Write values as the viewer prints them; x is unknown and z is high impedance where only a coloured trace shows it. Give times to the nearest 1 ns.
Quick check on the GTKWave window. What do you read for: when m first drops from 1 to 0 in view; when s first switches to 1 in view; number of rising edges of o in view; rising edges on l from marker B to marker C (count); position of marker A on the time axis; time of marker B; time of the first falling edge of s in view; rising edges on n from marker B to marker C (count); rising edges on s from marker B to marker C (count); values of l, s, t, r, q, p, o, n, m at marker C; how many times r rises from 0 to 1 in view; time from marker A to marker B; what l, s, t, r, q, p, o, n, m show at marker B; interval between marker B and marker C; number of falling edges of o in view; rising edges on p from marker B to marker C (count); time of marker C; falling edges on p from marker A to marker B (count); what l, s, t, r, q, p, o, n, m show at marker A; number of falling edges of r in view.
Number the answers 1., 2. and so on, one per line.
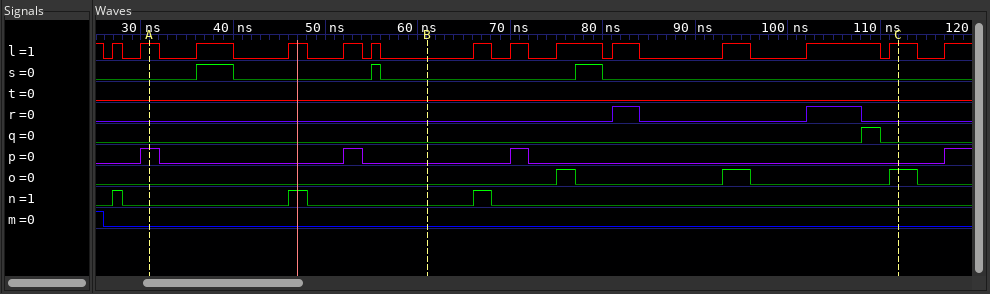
1. 26 ns
2. 36 ns
3. 3
4. 7
5. 31 ns
6. 61 ns
7. 40 ns
8. 1
9. 1
10. l=1, s=0, t=0, r=0, q=0, p=0, o=1, n=0, m=0
11. 2
12. 30 ns
13. l=0, s=0, t=0, r=0, q=0, p=0, o=0, n=0, m=0
14. 51 ns
15. 3
16. 1
17. 112 ns
18. 2
19. l=1, s=0, t=0, r=0, q=0, p=1, o=0, n=0, m=0
20. 2
